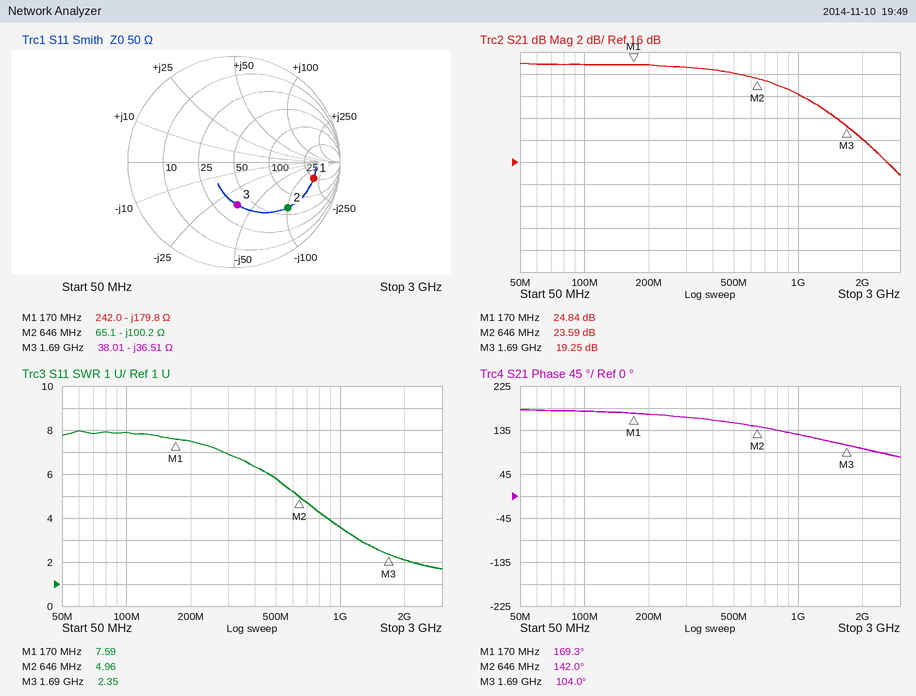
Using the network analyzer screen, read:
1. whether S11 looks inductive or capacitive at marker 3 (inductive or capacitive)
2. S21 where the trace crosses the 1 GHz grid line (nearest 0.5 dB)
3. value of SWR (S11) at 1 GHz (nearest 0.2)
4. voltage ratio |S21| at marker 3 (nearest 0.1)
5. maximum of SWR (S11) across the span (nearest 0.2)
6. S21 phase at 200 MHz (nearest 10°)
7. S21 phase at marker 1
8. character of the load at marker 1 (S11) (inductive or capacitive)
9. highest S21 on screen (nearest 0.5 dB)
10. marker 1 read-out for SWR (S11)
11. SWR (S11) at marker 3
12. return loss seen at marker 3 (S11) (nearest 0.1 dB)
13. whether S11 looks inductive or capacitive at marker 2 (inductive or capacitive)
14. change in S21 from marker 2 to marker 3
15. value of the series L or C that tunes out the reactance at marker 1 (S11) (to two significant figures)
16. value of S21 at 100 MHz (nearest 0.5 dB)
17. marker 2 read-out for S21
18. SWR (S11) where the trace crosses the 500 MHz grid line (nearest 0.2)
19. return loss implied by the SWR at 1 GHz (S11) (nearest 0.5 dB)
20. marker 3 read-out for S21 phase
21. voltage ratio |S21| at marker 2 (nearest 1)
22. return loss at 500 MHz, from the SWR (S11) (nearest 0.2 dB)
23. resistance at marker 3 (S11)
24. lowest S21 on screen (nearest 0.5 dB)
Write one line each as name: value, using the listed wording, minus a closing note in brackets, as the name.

whether S11 looks inductive or capacitive at marker 3: capacitive
S21 where the trace crosses the 1 GHz grid line: 22.0 dB
value of SWR (S11) at 1 GHz: 3.6
voltage ratio |S21| at marker 3: 9.2
maximum of SWR (S11) across the span: 8.0
S21 phase at 200 MHz: 170°
S21 phase at marker 1: 169.3°
character of the load at marker 1 (S11): capacitive
highest S21 on screen: 25.0 dB
marker 1 read-out for SWR: 7.59
SWR (S11) at marker 3: 2.35
return loss seen at marker 3 (S11): 7.9 dB
whether S11 looks inductive or capacitive at marker 2: capacitive
change in S21 from marker 2 to marker 3: -4.34 dB
value of the series L or C that tunes out the reactance at marker 1 (S11): 170 nH
value of S21 at 100 MHz: 25.0 dB
marker 2 read-out for S21: 23.59 dB
SWR (S11) where the trace crosses the 500 MHz grid line: 5.8
return loss implied by the SWR at 1 GHz (S11): 5.0 dB
marker 3 read-out for S21 phase: 104.0°
voltage ratio |S21| at marker 2: 15
return loss at 500 MHz, from the SWR (S11): 3.0 dB
resistance at marker 3: 38.01 Ω
lowest S21 on screen: 15.0 dB
